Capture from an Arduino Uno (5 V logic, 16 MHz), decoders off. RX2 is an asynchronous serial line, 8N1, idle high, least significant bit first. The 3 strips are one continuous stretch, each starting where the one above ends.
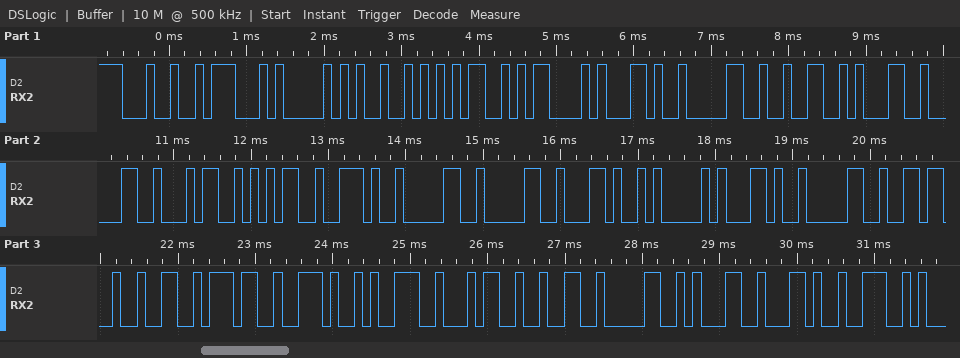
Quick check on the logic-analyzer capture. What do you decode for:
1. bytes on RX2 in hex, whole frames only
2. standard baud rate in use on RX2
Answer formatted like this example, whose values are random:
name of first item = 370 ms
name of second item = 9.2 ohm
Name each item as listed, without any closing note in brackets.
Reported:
bytes on RX2 in hex, whole frames only = 24 47 50 52 4D 43 2C 30 32 31 30 34 35 2E 30 30 2C 41 2C 30 36 32 37 2E 39 34 32 30 31 2C 4E
standard baud rate in use on RX2 = 9600 baud
